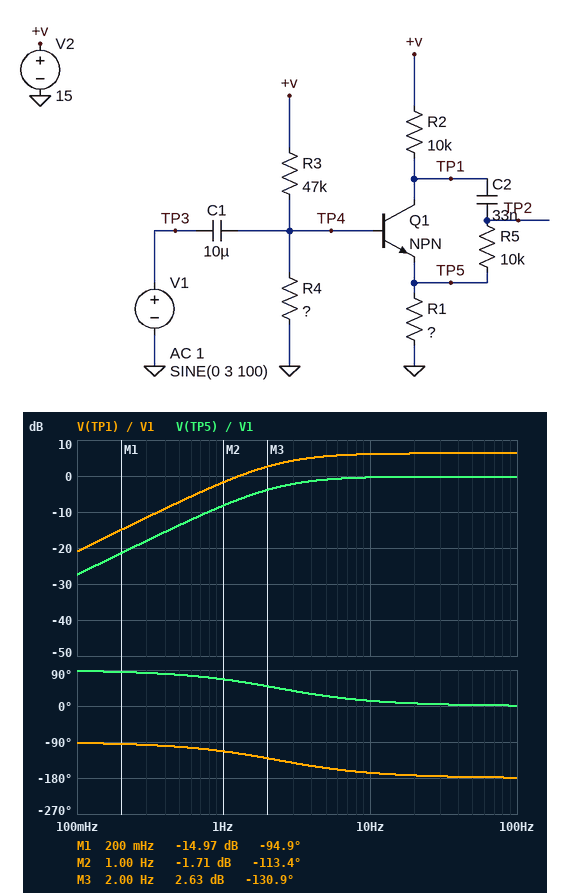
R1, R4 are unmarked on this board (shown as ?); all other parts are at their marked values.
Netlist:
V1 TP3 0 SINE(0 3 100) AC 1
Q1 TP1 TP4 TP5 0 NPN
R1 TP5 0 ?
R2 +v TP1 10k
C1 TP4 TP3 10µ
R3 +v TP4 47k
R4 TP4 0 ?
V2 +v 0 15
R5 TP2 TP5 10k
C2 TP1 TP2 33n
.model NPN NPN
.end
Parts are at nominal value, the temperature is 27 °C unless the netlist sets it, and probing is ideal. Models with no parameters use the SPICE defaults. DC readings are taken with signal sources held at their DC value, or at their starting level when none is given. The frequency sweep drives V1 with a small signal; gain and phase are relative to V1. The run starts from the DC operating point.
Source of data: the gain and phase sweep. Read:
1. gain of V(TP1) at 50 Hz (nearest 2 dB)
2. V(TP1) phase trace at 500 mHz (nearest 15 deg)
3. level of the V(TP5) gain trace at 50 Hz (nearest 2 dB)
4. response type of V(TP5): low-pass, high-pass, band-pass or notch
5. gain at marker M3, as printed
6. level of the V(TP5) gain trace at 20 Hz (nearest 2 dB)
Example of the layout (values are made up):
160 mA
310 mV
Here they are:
6 dB
-105 deg
0 dB
high-pass
2.63 dB
0 dB
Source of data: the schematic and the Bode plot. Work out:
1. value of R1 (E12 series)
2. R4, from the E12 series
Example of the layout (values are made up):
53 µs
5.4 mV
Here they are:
4.7 kΩ
8.2 kΩ
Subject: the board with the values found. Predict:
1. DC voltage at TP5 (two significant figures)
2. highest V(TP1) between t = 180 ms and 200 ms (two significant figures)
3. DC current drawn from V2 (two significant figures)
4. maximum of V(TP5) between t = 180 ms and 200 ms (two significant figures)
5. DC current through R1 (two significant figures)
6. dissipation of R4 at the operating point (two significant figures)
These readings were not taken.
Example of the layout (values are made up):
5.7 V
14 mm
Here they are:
1.5 V
15 V
580 µA
4.4 V
310 µA
590 µW
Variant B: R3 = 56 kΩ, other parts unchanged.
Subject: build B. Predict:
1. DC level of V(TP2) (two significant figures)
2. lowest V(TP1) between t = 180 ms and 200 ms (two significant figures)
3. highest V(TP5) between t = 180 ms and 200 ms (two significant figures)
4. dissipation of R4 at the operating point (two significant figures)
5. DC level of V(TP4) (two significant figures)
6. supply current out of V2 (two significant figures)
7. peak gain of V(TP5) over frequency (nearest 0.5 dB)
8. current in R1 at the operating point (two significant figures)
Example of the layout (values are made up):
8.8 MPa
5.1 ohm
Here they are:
1.2 V
6.3 V
4.1 V
440 µW
1.9 V
480 µA
0 dB
250 µA
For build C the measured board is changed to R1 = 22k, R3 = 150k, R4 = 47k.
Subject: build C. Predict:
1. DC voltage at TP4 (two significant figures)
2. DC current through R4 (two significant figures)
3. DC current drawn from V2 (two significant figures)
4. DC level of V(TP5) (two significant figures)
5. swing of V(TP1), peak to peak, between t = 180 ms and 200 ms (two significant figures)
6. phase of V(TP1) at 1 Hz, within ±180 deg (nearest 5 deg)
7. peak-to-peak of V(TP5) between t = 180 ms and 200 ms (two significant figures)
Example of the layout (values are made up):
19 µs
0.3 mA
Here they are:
3.5 V
75 µA
200 µA
2.8 V
2.5 V
-155 deg
5.5 V
